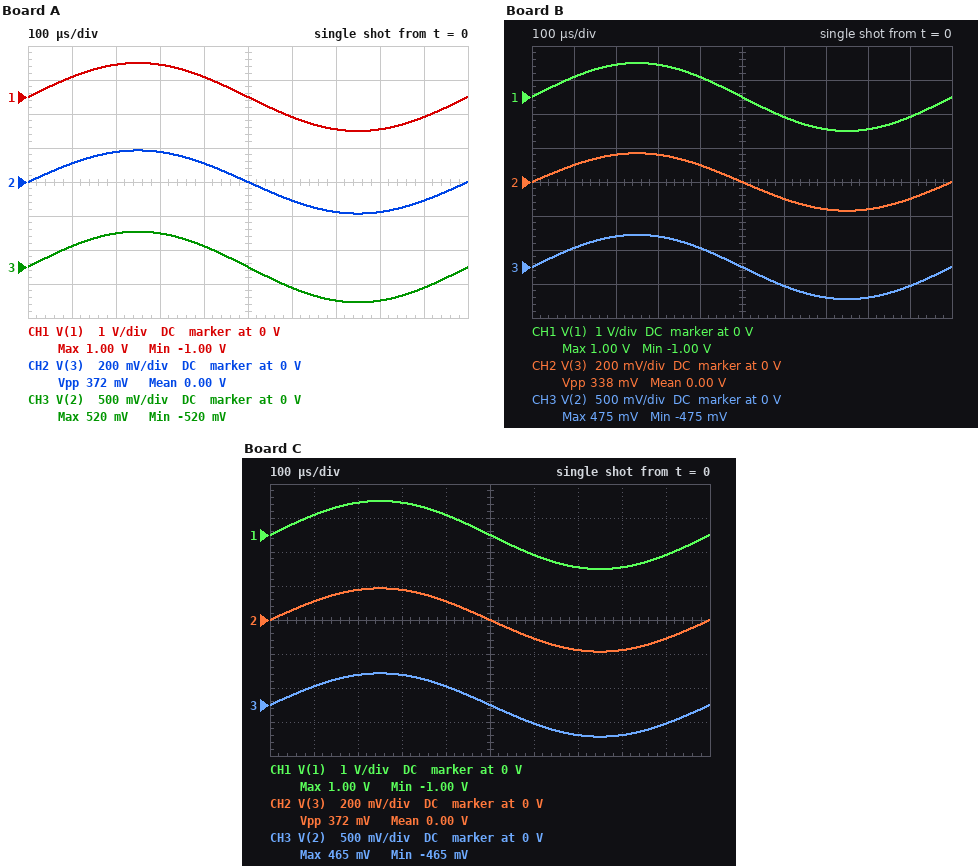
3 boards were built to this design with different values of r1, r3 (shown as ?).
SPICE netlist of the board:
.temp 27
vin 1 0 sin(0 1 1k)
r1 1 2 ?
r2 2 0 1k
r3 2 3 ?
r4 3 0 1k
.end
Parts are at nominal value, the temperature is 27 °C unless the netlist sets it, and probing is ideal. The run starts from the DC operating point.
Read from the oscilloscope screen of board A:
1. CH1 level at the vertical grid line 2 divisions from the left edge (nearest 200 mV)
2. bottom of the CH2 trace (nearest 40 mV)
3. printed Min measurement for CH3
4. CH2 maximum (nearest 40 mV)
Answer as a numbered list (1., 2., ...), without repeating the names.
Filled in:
1. 1.0 V
2. -200 mV
3. -520 mV
4. 200 mV
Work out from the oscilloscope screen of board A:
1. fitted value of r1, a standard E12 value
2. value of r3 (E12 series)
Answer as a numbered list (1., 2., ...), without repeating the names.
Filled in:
1. 680 Ω
2. 1.8 kΩ
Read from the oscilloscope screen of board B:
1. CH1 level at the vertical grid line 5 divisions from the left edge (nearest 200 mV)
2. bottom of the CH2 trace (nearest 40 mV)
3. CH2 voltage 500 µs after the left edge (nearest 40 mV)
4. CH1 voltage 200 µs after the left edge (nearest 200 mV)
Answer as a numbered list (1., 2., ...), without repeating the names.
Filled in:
1. 0 V
2. -160 mV
3. 0 V
4. 1.0 V
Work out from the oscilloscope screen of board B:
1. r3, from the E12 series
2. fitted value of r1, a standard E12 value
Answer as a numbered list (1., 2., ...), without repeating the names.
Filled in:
1. 1.8 kΩ
2. 820 Ω
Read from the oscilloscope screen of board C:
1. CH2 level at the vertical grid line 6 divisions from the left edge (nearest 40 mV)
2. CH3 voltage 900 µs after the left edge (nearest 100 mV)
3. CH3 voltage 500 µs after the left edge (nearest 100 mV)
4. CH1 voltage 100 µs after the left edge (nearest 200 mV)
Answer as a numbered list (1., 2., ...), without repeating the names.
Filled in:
1. -120 mV
2. -300 mV
3. 0 V
4. 600 mV
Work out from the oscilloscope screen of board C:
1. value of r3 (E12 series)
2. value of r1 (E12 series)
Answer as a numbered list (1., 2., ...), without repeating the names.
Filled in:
1. 1.5 kΩ
2. 820 Ω
